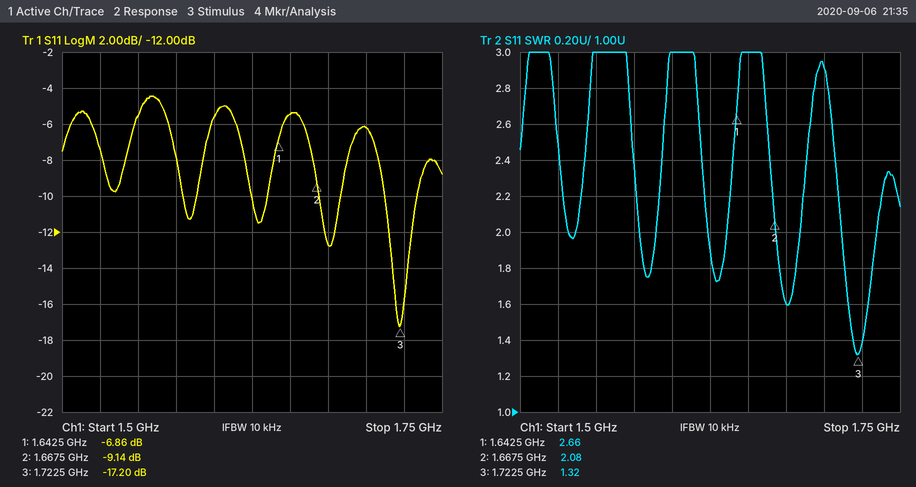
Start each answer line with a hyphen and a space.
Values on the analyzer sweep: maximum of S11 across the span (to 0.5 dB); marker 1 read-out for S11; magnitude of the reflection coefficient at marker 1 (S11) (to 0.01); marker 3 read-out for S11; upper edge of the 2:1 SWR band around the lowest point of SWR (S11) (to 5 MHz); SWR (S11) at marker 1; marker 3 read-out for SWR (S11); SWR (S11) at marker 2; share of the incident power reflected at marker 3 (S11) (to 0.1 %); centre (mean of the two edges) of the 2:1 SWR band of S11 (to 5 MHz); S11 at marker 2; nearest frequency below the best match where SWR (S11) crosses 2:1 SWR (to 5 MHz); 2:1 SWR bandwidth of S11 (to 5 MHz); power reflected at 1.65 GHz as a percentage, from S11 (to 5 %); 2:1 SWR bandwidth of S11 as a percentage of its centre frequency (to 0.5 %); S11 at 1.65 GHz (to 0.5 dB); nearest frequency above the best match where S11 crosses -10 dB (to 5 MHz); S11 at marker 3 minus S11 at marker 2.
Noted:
- -4.5 dB
- -6.86 dB
- 0.45
- -17.20 dB
- 1.735 GHz
- 2.66
- 1.32
- 2.08
- 1.9 %
- 1.725 GHz
- -9.14 dB
- 1.710 GHz
- 25 MHz
- 30 %
- 1.5 %
- -5.5 dB
- 1.735 GHz
- -8.06 dB
